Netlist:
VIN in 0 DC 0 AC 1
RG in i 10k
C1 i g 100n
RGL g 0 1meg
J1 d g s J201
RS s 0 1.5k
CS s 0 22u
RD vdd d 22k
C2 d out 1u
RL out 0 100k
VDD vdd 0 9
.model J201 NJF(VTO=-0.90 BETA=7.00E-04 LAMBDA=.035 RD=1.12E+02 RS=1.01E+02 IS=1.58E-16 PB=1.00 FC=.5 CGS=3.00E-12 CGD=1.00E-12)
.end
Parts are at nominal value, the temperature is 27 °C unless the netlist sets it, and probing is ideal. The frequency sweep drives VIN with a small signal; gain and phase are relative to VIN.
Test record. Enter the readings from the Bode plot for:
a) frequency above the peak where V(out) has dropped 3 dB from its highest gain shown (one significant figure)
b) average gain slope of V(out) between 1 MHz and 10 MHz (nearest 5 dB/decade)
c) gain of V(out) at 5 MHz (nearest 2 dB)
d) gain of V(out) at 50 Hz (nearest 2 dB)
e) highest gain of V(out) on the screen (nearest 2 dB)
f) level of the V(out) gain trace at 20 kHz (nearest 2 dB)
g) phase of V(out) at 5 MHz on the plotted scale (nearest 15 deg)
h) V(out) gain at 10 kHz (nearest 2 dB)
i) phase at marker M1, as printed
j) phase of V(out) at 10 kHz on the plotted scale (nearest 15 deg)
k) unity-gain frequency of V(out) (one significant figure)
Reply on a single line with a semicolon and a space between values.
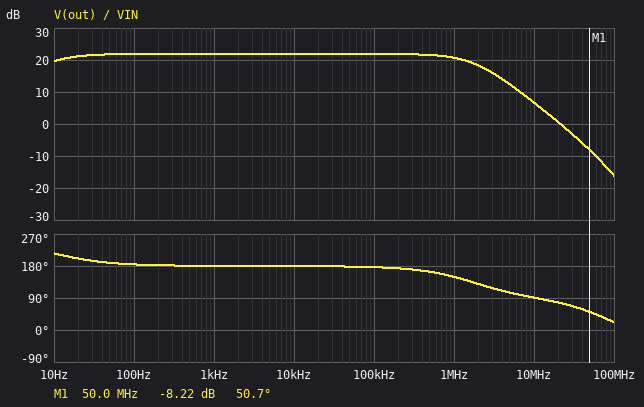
2 MHz; -15 dB/decade; 12 dB; 22 dB; 22 dB; 22 dB; 105 deg; 22 dB; 50.7 deg; 180 deg; 20 MHz
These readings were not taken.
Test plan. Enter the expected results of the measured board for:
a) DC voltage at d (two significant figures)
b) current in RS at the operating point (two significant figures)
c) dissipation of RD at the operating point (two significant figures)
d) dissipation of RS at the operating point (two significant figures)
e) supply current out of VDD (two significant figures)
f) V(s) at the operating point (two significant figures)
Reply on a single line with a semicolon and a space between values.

4.0 V; 230 µA; 1.1 mW; 77 µW; 230 µA; 340 mV
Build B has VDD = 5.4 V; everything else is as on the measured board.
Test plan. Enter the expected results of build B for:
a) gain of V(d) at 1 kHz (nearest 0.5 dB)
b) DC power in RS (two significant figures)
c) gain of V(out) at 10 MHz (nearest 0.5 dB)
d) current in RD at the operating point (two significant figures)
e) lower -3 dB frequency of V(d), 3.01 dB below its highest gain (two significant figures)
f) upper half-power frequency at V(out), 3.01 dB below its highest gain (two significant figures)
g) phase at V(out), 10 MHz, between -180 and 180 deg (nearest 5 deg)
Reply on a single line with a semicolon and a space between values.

6.5 dB; 66 µW; -4.0 dB; 210 µA; 2.4 Hz; 3.1 MHz; 95 deg
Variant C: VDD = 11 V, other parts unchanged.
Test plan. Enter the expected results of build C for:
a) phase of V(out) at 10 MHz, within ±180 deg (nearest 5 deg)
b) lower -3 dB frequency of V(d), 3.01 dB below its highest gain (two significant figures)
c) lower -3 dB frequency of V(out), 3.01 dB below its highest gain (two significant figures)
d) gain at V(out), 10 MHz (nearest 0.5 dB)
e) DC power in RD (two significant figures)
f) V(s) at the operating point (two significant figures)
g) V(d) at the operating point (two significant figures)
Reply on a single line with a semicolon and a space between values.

95 deg; 7.8 Hz; 8.2 Hz; 8.0 dB; 1.2 mW; 350 mV; 5.9 V
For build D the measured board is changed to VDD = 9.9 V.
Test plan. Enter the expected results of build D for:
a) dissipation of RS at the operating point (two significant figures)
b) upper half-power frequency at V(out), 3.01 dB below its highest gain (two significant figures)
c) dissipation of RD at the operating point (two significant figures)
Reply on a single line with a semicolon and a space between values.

79 µW; 1.9 MHz; 1.2 mW
